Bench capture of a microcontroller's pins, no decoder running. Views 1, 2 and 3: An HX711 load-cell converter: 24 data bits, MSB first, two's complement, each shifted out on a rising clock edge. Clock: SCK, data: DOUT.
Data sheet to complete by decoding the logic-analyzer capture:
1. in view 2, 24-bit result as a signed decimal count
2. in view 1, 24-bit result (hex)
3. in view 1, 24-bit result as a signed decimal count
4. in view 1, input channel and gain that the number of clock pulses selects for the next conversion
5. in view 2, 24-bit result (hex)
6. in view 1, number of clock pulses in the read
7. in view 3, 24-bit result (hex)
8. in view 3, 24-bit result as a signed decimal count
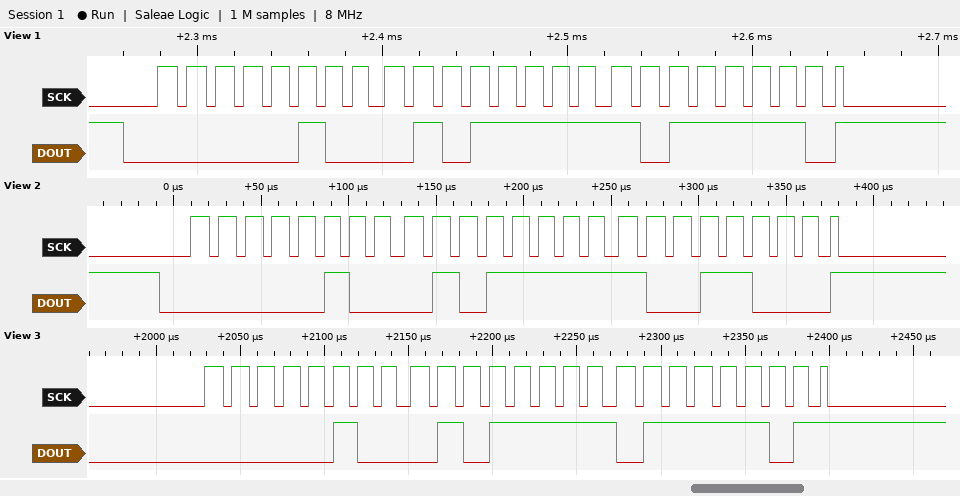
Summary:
286616
0x045FBE
286654
channel A, gain 128
0x045F98
25
0x045F7D
286589
